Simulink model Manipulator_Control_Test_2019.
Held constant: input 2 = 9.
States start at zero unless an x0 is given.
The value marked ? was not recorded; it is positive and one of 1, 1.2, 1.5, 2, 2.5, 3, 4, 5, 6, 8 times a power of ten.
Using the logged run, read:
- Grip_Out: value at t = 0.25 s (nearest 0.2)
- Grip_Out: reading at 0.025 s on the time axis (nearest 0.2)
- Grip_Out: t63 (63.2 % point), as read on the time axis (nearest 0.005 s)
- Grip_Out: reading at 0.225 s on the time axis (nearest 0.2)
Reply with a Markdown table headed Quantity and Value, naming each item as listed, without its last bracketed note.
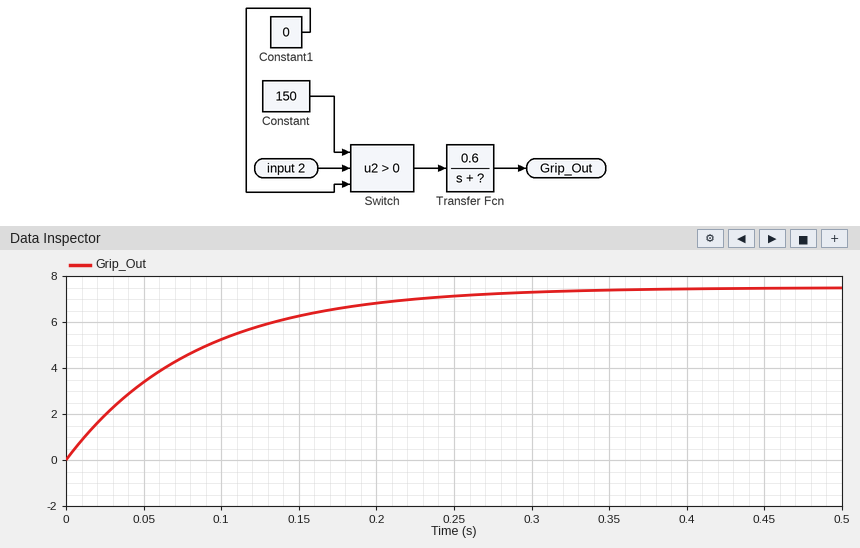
| Quantity | Value |
|---|---|
| Grip_Out: value at t = 0.25 s | 7.2 |
| Grip_Out: reading at 0.025 s on the time axis | 2.0 |
| Grip_Out: t63 (63.2 % point), as read on the time axis | 0.085 s |
| Grip_Out: reading at 0.225 s on the time axis | 7.0 |
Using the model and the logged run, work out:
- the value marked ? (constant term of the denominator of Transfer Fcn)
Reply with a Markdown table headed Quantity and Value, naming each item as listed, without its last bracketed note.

| Quantity | Value |
|---|---|
| the value marked ? | 12 |
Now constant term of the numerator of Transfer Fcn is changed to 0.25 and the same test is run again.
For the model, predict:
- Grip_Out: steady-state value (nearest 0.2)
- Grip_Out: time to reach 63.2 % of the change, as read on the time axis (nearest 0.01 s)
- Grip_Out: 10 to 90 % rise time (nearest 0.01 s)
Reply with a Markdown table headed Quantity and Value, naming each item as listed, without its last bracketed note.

| Quantity | Value |
|---|---|
| Grip_Out: steady-state value | 3.2 |
| Grip_Out: time to reach 63.2 % of the change, as read on the time axis | 0.08 s |
| Grip_Out: 10 to 90 % rise time | 0.18 s |
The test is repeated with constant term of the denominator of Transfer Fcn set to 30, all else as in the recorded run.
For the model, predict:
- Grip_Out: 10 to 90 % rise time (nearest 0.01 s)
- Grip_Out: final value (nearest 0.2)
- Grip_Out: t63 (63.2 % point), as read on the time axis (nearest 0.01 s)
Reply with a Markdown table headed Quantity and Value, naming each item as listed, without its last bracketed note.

| Quantity | Value |
|---|---|
| Grip_Out: 10 to 90 % rise time | 0.07 s |
| Grip_Out: final value | 3.0 |
| Grip_Out: t63 (63.2 % point), as read on the time axis | 0.03 s |
